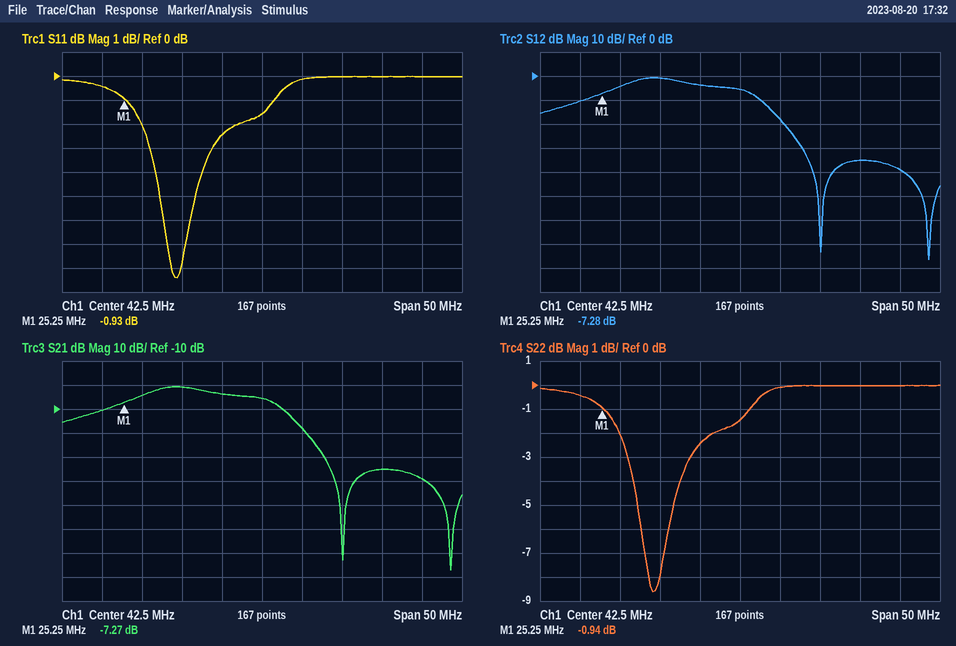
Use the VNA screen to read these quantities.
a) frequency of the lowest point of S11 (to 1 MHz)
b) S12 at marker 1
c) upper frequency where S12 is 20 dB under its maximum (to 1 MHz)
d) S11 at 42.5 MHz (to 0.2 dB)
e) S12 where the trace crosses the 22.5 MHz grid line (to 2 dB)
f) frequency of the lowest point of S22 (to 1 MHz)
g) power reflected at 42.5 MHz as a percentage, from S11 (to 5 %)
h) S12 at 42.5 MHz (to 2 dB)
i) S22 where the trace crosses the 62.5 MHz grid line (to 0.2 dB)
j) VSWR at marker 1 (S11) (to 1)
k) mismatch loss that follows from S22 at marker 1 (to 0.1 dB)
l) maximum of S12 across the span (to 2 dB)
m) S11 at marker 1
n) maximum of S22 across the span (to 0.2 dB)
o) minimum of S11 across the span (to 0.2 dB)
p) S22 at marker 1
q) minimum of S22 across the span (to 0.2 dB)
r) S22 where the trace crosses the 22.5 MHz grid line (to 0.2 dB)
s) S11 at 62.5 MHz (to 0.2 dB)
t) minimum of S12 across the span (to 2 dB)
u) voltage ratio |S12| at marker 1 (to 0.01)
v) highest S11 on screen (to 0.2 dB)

32 MHz
-7.28 dB
48 MHz
-1.6 dB
-10 dB
32 MHz
70 %
-6 dB
0.0 dB
19
7.1 dB
0 dB
-0.93 dB
0.0 dB
-8.4 dB
-0.94 dB
-8.6 dB
-0.4 dB
0.0 dB
-76 dB
0.43
0.0 dB
